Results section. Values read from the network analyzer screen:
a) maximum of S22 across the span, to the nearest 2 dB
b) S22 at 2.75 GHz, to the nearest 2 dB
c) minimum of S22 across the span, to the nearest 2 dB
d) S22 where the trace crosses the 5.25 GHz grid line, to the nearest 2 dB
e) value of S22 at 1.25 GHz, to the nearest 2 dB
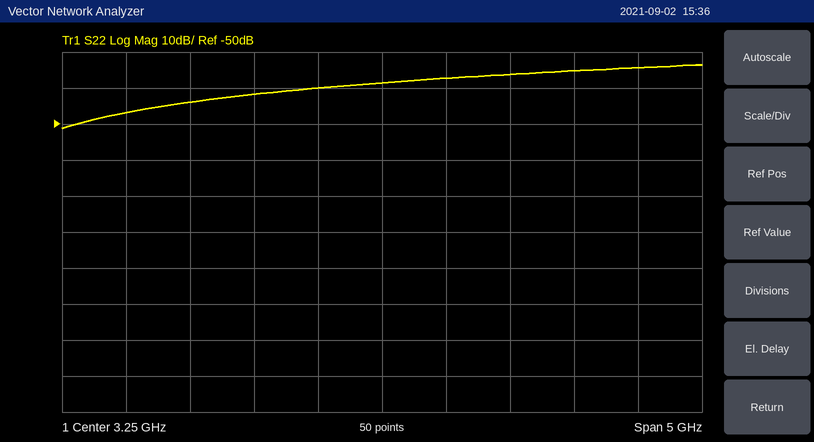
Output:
-34 dB
-40 dB
-52 dB
-34 dB
-46 dB
